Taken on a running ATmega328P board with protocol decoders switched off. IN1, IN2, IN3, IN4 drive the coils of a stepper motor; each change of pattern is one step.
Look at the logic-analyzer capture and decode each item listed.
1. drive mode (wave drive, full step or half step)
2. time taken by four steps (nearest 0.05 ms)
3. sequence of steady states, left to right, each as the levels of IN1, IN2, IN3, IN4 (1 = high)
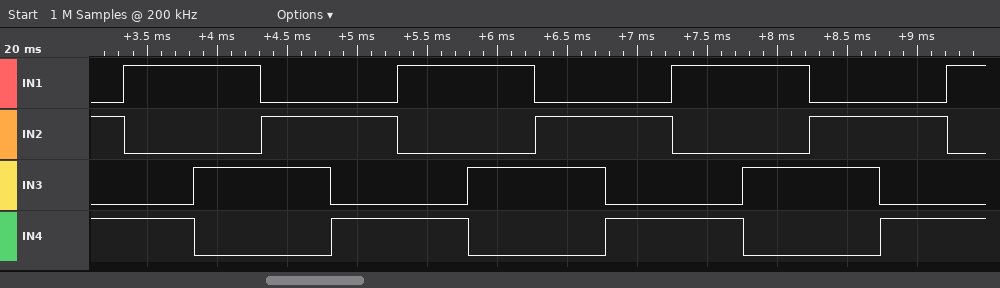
full step
1.95 ms
0101 1001 1010 0110 0101 1001 1010 0110 0101 1001 1010 0110 0101 1001
